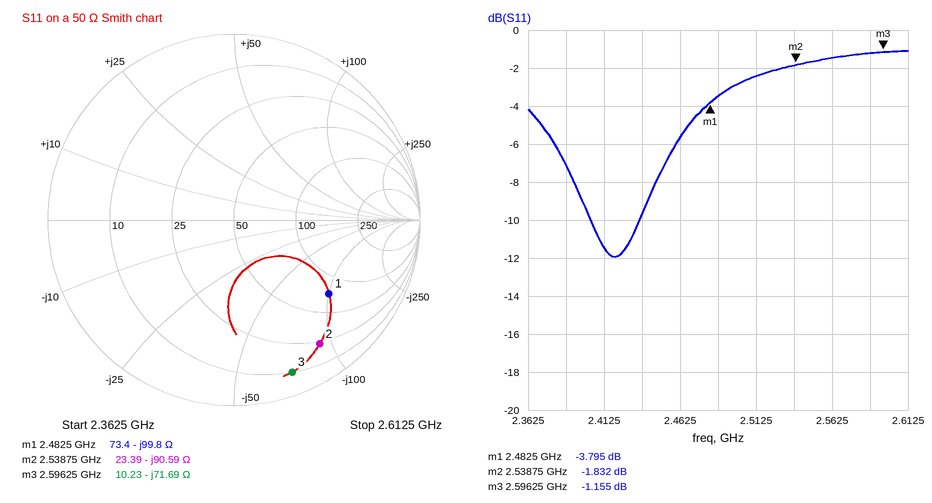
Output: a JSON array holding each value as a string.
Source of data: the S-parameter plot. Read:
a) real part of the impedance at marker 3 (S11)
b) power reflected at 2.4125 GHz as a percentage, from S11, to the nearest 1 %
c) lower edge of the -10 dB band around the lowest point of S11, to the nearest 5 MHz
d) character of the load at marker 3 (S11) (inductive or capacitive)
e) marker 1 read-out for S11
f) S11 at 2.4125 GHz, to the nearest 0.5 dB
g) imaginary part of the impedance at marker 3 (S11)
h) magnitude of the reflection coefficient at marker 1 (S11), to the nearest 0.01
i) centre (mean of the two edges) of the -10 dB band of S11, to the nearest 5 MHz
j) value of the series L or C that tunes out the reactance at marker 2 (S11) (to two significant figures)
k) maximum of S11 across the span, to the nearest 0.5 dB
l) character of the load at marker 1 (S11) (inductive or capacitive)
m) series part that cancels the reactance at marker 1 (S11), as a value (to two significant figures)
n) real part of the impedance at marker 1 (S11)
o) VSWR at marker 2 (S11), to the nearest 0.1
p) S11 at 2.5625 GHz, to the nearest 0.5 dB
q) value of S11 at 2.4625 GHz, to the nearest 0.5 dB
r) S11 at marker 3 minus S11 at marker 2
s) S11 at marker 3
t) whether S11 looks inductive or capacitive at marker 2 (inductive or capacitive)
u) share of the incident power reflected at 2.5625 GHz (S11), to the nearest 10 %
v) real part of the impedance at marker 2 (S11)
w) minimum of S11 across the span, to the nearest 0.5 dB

["10.23 Ω", "7 %", "2.405 GHz", "capacitive", "-3.795 dB", "-11.5 dB", "-71.69 Ω", "0.65", "2.420 GHz", "5.7 nH", "-1.0 dB", "capacitive", "6.4 nH", "73.4 Ω", "9.5", "-1.5 dB", "-5.5 dB", "0.677 dB", "-1.155 dB", "capacitive", "70 %", "23.39 Ω", "-12.0 dB"]
